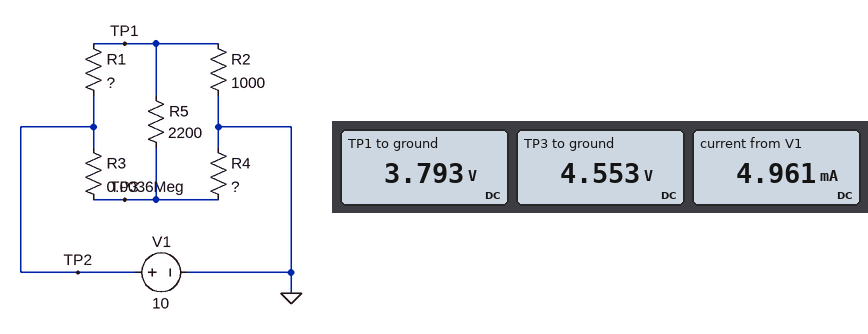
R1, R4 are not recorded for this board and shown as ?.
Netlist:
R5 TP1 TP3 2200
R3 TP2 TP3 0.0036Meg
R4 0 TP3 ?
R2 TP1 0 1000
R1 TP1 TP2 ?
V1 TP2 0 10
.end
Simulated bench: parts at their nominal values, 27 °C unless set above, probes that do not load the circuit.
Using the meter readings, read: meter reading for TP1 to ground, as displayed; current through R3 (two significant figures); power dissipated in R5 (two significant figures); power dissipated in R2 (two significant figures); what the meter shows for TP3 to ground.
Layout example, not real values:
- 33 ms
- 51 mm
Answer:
- 3.793 V
- 1.5 mA
- 260 µW
- 14 mW
- 4.553 V
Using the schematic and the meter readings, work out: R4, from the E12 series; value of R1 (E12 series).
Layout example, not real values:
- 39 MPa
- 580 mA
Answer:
- 3.9 kΩ
- 1.8 kΩ
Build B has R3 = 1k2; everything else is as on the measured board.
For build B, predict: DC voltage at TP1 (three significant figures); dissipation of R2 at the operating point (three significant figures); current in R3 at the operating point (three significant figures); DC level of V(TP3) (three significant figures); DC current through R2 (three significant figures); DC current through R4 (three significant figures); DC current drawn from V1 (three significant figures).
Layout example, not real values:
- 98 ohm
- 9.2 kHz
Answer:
- 4.27 V
- 18.2 mW
- 2.79 mA
- 6.65 V
- 4.27 mA
- 1.71 mA
- 5.97 mA
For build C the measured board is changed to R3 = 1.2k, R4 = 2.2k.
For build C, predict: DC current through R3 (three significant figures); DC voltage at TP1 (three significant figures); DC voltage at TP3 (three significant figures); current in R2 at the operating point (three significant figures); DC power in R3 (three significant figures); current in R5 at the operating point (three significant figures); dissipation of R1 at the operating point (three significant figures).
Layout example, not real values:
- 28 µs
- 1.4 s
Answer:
- 3.46 mA
- 4.09 V
- 5.85 V
- 4.09 mA
- 14.4 mW
- 801 µA
- 19.4 mW
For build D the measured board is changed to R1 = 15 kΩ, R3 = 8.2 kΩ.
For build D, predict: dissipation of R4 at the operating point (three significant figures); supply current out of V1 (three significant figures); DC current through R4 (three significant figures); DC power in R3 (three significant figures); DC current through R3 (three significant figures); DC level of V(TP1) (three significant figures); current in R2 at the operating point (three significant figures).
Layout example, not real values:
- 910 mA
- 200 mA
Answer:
- 1.06 mW
- 1.57 mA
- 522 µA
- 7.74 mW
- 971 µA
- 1.05 V
- 1.05 mA
